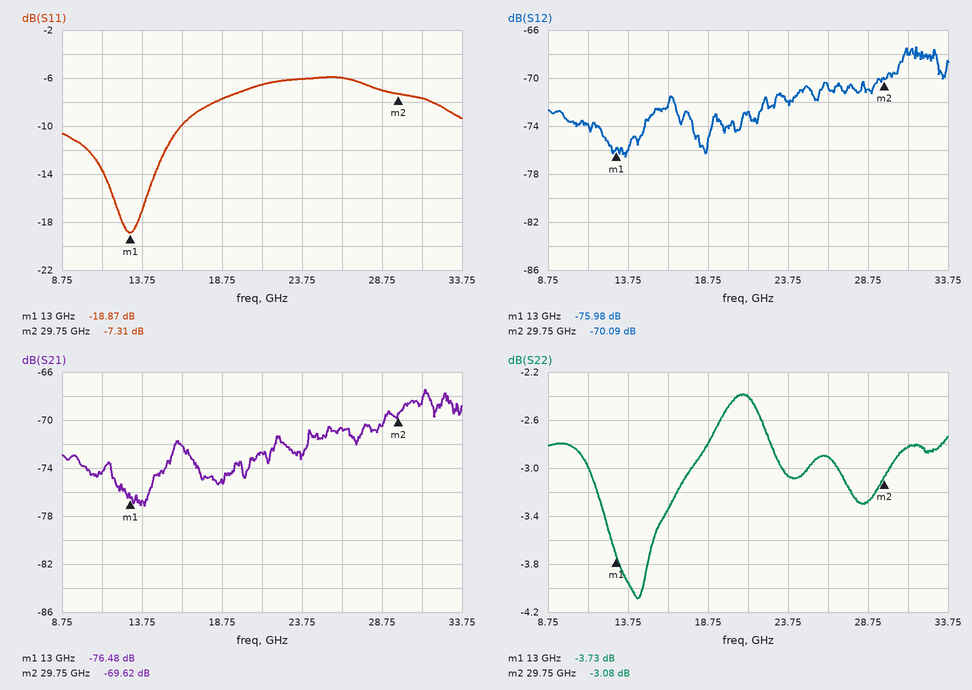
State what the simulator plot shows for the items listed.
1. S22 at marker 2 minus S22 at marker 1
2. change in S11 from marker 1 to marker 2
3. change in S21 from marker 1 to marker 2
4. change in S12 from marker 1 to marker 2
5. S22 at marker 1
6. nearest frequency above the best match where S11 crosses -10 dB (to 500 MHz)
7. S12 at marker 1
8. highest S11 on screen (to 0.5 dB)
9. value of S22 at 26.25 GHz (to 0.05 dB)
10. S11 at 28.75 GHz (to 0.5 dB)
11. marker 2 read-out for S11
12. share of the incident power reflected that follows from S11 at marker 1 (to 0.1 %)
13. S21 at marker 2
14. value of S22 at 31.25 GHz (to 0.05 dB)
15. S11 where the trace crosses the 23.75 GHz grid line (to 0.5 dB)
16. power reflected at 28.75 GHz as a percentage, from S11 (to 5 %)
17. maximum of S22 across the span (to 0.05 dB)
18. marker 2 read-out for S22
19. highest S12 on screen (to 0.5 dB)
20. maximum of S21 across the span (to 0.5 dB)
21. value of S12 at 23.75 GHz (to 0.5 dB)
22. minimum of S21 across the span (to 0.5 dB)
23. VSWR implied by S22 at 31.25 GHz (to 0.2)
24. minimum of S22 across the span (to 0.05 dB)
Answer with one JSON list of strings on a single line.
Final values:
["0.65 dB", "11.56 dB", "6.86 dB", "5.89 dB", "-3.73 dB", "16.0 GHz", "-75.98 dB", "-6.0 dB", "-2.90 dB", "-7.0 dB", "-7.31 dB", "1.3 %", "-69.62 dB", "-2.80 dB", "-6.0 dB", "20 %", "-2.40 dB", "-3.08 dB", "-67.5 dB", "-67.5 dB", "-72.0 dB", "-77.0 dB", "6.2", "-4.10 dB"]
